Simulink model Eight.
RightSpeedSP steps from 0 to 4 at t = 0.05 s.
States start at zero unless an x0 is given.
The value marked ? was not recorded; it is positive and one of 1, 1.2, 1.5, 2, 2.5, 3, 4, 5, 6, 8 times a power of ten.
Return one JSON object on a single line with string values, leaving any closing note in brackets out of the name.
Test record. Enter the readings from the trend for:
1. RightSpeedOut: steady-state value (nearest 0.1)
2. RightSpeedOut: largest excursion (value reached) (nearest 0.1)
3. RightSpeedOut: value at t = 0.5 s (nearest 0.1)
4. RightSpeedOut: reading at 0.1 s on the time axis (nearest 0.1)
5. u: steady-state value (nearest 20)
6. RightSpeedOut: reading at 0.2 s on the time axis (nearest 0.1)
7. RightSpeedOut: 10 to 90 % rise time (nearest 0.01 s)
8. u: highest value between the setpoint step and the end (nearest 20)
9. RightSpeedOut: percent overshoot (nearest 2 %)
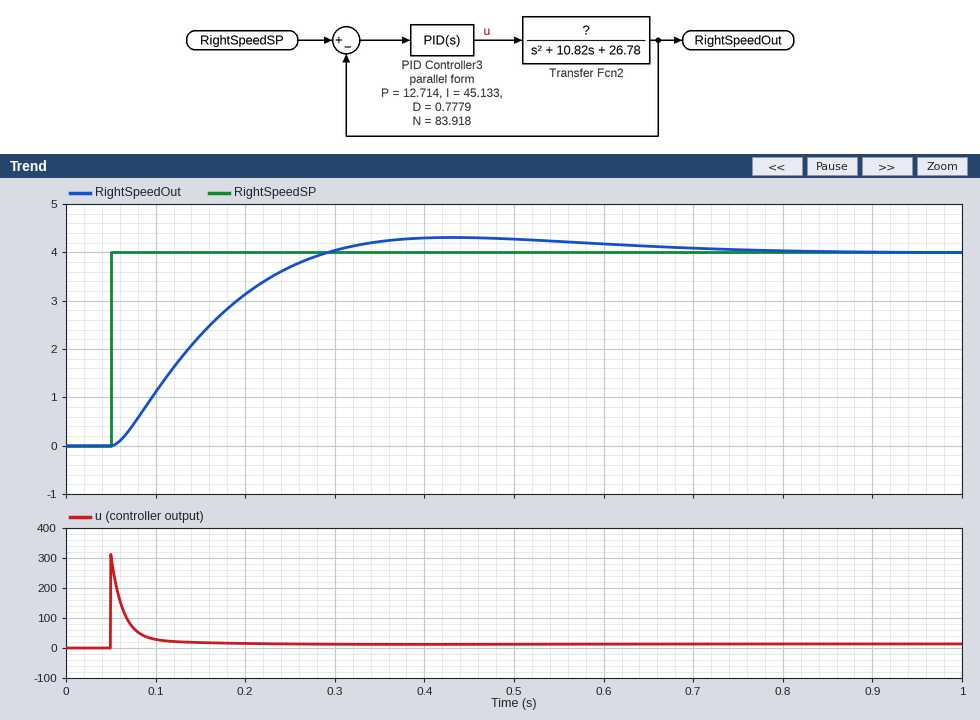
{"RightSpeedOut: steady-state value": "4.0", "RightSpeedOut: largest excursion (value reached)": "4.3", "RightSpeedOut: value at t = 0.5 s": "4.3", "RightSpeedOut: reading at 0.1 s on the time axis": "1.1", "u: steady-state value": "20", "RightSpeedOut: reading at 0.2 s on the time axis": "3.1", "RightSpeedOut: 10 to 90 % rise time": "0.17 s", "u: highest value between the setpoint step and the end": "320", "RightSpeedOut: percent overshoot": "8 %"}
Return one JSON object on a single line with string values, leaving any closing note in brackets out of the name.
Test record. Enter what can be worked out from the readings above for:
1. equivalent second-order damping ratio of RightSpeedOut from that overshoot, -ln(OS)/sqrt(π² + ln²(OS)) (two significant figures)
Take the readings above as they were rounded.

{"equivalent second-order damping ratio of RightSpeedOut from that overshoot, -ln(OS)/sqrt(π² + ln²(OS))": "0.63"}
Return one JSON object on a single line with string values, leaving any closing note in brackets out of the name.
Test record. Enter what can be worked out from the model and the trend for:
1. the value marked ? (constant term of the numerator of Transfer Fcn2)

{"the value marked ?": "8"}
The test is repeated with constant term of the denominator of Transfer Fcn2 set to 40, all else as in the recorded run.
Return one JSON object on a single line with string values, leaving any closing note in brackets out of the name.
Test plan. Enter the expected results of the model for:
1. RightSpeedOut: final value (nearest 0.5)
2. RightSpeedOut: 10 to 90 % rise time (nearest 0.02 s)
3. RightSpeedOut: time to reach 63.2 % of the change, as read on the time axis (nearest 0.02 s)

{"RightSpeedOut: final value": "4.0", "RightSpeedOut: 10 to 90 % rise time": "0.18 s", "RightSpeedOut: time to reach 63.2 % of the change, as read on the time axis": "0.16 s"}
